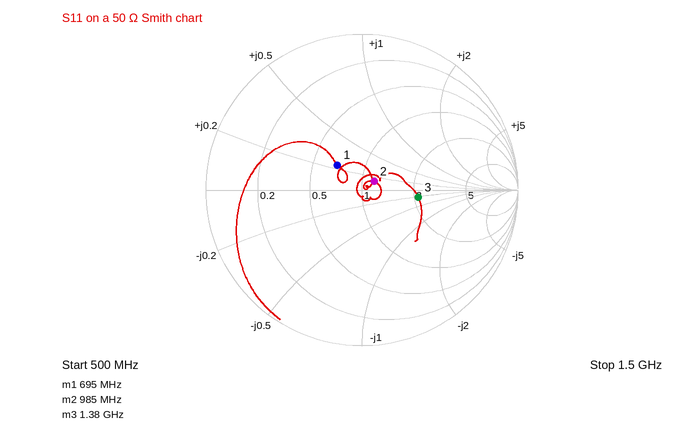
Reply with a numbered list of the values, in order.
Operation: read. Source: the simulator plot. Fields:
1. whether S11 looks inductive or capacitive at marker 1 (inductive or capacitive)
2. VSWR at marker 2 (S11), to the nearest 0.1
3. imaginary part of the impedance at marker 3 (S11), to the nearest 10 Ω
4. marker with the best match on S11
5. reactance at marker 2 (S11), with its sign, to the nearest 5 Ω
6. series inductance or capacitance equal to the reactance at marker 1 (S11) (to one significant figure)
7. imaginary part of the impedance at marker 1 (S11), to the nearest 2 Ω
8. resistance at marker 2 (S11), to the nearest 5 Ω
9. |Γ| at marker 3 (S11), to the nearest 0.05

1. inductive
2. 1.2
3. -10 Ω
4. marker 2
5. +5 Ω
6. 3 nH
7. +12 Ω
8. 60 Ω
9. 0.35
